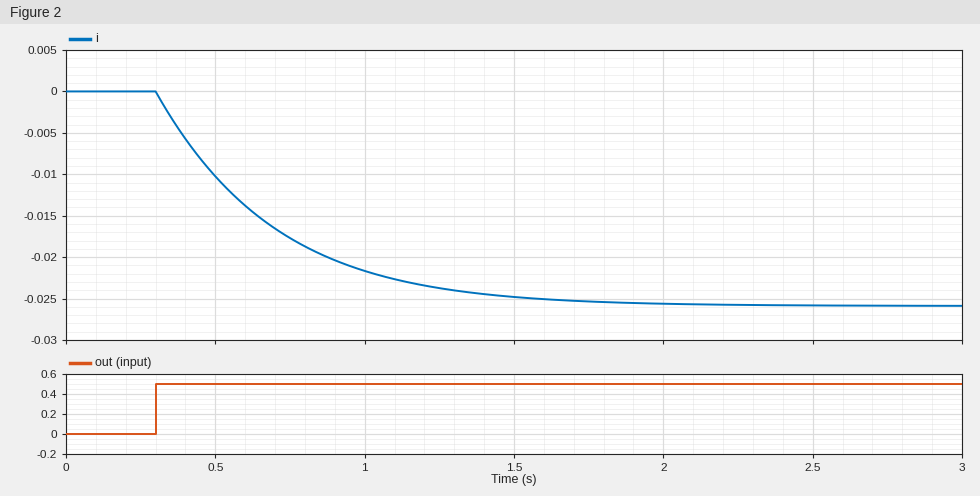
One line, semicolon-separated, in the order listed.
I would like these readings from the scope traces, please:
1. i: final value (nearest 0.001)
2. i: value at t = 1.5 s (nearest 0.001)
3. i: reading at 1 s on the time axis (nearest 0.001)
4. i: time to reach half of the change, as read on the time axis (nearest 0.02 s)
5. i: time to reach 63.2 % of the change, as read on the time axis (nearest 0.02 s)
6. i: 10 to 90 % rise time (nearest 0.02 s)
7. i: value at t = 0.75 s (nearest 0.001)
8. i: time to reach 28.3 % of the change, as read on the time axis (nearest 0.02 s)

-0.026; -0.025; -0.022; 0.58 s; 0.70 s; 0.84 s; -0.018; 0.44 s
